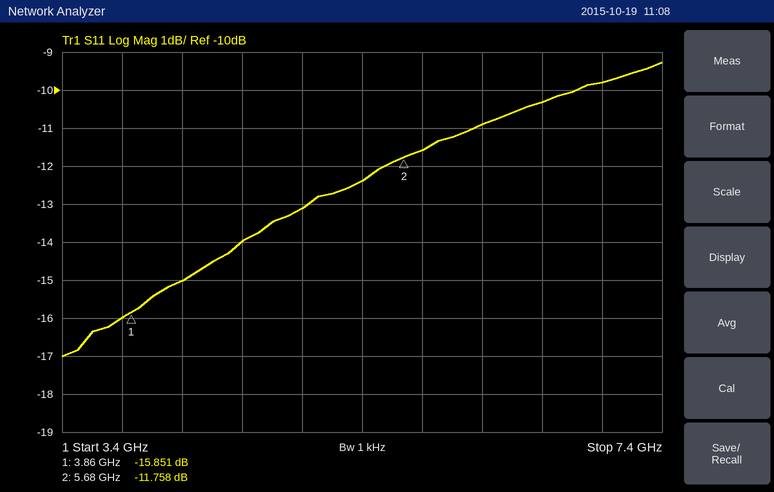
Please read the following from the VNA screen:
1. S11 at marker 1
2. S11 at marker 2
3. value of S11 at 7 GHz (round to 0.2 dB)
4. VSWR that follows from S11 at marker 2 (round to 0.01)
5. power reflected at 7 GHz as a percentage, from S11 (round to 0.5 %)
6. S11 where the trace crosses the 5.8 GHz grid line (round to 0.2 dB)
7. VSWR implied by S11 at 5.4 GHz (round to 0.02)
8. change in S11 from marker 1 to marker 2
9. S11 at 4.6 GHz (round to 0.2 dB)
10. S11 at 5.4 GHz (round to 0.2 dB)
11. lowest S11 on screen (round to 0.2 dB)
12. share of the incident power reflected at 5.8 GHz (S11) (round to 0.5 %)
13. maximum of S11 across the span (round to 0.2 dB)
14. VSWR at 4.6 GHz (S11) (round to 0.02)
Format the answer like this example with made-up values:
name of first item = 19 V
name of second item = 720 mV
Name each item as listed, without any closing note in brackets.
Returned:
S11 at marker 1 = -15.851 dB
S11 at marker 2 = -11.758 dB
value of S11 at 7 GHz = -9.8 dB
VSWR that follows from S11 at marker 2 = 1.70
power reflected at 7 GHz as a percentage, from S11 = 10.5 %
S11 where the trace crosses the 5.8 GHz grid line = -11.6 dB
VSWR implied by S11 at 5.4 GHz = 1.64
change in S11 from marker 1 to marker 2 = 4.093 dB
S11 at 4.6 GHz = -14.0 dB
S11 at 5.4 GHz = -12.4 dB
lowest S11 on screen = -17.0 dB
share of the incident power reflected at 5.8 GHz (S11) = 7.0 %
maximum of S11 across the span = -9.2 dB
VSWR at 4.6 GHz (S11) = 1.50
